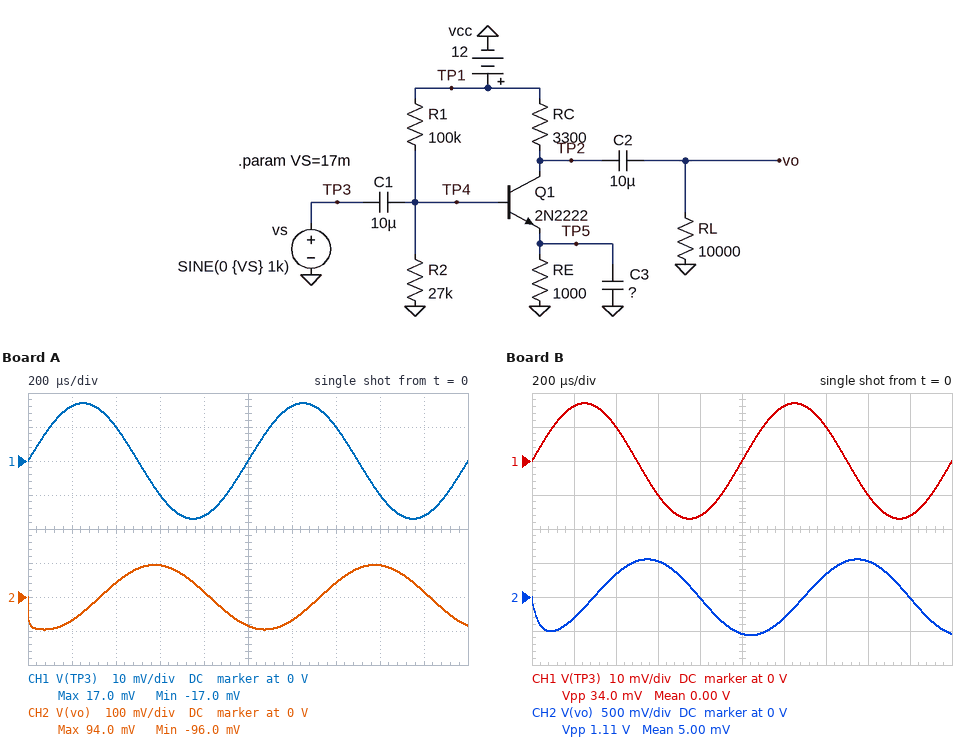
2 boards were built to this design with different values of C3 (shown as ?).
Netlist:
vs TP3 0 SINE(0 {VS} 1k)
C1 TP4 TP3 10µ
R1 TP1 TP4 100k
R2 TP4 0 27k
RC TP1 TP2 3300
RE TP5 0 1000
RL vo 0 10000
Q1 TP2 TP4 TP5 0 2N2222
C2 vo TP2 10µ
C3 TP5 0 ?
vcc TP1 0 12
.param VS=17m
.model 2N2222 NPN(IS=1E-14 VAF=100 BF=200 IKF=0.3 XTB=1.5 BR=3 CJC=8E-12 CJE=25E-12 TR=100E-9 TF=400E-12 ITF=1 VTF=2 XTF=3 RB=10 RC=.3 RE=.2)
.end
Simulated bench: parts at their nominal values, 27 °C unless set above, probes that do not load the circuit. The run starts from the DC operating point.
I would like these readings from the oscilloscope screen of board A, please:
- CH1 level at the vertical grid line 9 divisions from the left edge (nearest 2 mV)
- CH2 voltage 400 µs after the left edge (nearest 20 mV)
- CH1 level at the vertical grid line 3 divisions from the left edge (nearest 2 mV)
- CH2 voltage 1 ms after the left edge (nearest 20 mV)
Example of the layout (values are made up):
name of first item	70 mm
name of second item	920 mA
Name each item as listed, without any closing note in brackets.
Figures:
CH1 level at the vertical grid line 9 divisions from the left edge	-16 mV
CH2 voltage 400 µs after the left edge	40 mV
CH1 level at the vertical grid line 3 divisions from the left edge	-10 mV
CH2 voltage 1 ms after the left edge	-80 mV
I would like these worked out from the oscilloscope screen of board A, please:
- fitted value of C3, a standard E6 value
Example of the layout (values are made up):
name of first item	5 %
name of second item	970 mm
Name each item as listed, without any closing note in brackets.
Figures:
fitted value of C3, a standard E6 value	330 nF
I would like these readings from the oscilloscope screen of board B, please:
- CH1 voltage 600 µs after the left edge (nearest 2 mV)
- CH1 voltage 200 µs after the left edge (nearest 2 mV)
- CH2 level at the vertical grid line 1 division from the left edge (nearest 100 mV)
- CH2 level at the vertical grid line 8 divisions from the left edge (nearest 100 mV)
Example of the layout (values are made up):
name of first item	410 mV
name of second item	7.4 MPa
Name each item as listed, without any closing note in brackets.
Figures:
CH1 voltage 600 µs after the left edge	-10 mV
CH1 voltage 200 µs after the left edge	16 mV
CH2 level at the vertical grid line 1 division from the left edge	-300 mV
CH2 level at the vertical grid line 8 divisions from the left edge	500 mV
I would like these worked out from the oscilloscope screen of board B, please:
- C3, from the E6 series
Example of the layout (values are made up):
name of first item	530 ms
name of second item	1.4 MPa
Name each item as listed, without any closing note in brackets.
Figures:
C3, from the E6 series	2.2 µF
